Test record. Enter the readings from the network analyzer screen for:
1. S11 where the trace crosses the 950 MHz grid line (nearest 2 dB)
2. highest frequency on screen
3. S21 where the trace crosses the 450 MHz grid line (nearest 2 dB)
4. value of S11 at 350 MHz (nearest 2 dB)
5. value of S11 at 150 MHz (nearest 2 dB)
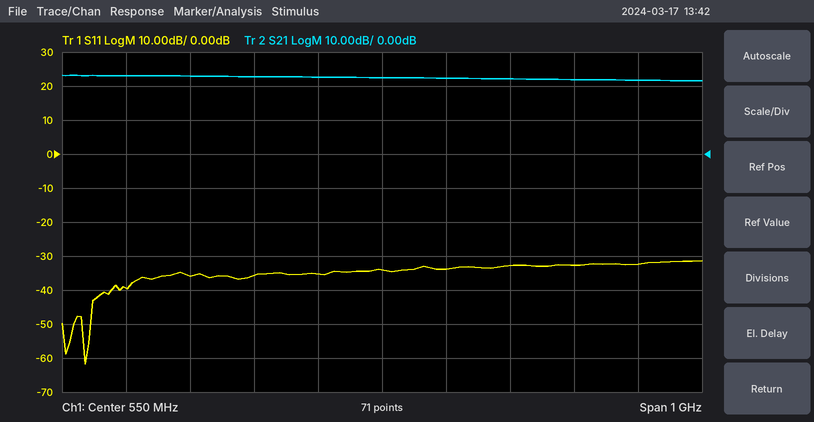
-32 dB
1.05 GHz
22 dB
-36 dB
-40 dB
